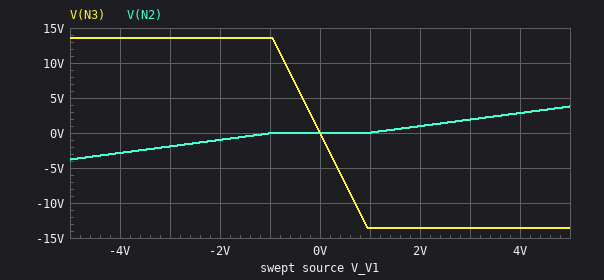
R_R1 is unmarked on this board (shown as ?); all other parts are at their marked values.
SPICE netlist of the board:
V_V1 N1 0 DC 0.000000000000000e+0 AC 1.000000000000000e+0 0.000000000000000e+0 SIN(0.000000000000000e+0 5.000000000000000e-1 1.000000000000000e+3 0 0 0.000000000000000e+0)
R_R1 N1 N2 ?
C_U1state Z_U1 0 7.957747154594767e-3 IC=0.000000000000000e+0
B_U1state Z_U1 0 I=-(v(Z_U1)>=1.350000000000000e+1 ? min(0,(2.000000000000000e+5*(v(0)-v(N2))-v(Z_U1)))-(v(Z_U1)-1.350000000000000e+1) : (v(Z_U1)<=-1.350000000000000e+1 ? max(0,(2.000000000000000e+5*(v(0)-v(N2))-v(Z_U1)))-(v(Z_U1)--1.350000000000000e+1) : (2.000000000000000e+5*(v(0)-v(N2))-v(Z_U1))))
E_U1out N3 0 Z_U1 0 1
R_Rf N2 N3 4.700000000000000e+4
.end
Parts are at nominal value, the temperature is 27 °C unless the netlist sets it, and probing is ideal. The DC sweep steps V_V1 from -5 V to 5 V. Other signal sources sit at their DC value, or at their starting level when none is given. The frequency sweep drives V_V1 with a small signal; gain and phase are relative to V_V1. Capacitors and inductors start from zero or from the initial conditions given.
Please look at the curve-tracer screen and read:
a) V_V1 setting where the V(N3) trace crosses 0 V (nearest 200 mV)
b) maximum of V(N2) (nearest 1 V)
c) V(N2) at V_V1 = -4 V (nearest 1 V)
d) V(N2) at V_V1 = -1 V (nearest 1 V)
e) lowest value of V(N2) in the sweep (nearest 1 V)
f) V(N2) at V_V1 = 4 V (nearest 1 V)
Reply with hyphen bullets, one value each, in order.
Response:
- 0 V
- 4 V
- -3 V
- 0 V
- -4 V
- 3 V
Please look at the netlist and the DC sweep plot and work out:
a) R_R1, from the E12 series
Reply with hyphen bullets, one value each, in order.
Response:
- 3.3 kΩ
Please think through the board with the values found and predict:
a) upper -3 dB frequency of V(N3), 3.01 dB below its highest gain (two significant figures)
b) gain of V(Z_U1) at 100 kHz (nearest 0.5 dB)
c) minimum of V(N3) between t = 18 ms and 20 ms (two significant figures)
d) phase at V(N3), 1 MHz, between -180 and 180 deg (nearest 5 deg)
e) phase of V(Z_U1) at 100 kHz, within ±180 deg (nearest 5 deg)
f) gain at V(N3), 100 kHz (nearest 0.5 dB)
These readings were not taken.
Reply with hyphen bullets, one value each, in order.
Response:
- 260 kHz
- 22.5 dB
- -7.1 V
- 105 deg
- 160 deg
- 22.5 dB
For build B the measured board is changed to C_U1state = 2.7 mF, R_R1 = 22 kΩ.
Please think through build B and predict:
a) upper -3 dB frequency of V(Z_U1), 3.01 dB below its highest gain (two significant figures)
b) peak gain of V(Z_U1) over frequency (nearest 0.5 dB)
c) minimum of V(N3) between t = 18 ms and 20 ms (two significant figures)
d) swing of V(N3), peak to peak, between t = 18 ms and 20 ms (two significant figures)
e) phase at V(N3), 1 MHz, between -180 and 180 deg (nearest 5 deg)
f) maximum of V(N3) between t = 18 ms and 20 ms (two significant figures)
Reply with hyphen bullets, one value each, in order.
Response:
- 3.8 MHz
- 6.5 dB
- -1.1 V
- 2.1 V
- 165 deg
- 1.1 V
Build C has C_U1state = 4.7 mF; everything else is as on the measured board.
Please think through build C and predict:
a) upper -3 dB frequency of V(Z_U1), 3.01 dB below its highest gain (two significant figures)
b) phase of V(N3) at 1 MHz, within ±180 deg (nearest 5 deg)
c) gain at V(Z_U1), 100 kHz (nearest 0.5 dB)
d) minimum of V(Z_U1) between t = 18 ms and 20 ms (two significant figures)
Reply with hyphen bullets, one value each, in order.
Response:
- 440 kHz
- 115 deg
- 23.0 dB
- -7.1 V
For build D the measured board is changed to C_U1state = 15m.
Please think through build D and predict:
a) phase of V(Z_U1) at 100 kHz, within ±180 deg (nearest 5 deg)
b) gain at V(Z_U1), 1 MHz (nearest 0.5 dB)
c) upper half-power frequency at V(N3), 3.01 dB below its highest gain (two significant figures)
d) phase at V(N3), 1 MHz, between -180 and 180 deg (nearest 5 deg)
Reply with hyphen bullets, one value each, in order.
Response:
- 145 deg
- 6.0 dB
- 140 kHz
- 100 deg
